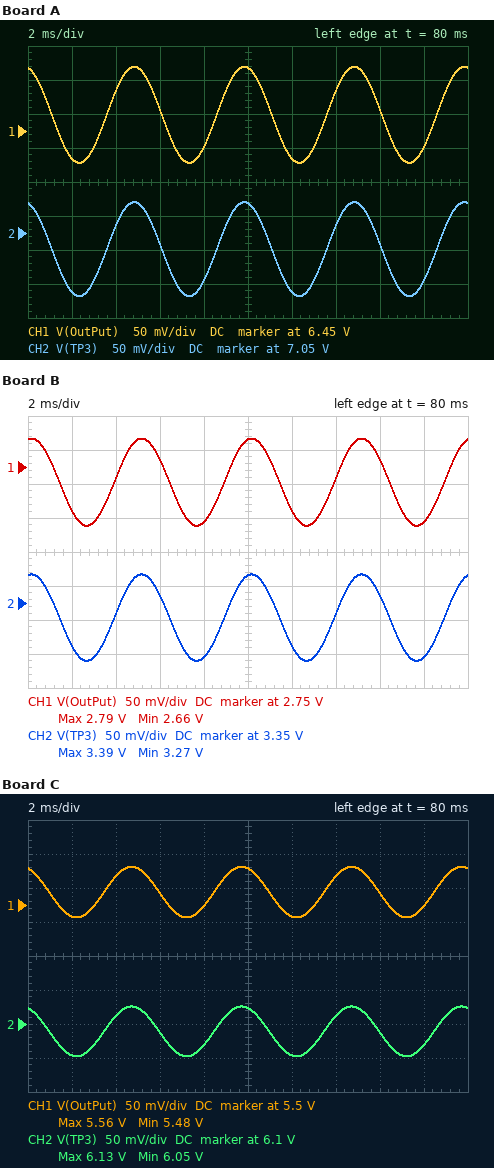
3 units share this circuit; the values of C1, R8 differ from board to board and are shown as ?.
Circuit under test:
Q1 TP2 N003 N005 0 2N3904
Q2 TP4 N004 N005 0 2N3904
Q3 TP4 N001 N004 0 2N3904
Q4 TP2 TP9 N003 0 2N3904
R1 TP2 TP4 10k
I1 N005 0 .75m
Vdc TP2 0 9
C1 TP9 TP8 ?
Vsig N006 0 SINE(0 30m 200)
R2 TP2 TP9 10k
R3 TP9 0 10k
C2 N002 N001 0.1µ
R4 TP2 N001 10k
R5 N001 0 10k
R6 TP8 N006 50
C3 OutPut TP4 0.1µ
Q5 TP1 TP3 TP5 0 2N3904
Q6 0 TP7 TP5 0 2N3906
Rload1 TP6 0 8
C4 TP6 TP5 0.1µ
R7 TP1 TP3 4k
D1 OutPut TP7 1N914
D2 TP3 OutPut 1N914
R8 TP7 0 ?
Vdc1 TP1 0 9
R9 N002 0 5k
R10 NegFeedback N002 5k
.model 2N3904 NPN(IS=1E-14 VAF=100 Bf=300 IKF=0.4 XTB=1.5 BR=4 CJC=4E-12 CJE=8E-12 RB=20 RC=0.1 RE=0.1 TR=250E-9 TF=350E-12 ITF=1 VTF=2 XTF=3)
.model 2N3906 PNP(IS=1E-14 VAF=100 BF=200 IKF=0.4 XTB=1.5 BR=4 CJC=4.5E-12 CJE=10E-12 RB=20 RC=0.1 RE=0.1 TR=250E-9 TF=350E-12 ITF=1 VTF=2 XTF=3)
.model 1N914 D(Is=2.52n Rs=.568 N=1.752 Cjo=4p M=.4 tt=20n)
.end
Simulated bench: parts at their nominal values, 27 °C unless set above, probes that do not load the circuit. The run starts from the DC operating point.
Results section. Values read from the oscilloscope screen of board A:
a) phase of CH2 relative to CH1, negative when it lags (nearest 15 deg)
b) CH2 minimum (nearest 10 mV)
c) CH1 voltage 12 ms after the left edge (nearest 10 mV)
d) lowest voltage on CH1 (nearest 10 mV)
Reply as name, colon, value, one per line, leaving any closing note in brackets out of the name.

phase of CH2 relative to CH1, negative when it lags: 0 deg
CH2 minimum: 6.96 V
CH1 voltage 12 ms after the left edge: 6.41 V
lowest voltage on CH1: 6.40 V
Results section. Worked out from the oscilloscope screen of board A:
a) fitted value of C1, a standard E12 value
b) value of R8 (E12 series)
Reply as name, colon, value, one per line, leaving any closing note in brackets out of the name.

fitted value of C1, a standard E12 value: 56 nF
value of R8: 12 kΩ
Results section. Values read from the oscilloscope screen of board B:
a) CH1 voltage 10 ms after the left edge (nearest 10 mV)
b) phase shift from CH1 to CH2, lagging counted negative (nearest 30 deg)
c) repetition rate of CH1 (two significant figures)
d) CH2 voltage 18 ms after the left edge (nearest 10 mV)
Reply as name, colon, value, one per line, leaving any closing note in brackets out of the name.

CH1 voltage 10 ms after the left edge: 2.79 V
phase shift from CH1 to CH2, lagging counted negative: 0 deg
repetition rate of CH1: 200 Hz
CH2 voltage 18 ms after the left edge: 3.27 V
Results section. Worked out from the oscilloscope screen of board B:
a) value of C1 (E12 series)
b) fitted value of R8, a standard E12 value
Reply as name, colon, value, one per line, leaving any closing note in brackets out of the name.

value of C1: 180 nF
fitted value of R8, a standard E12 value: 1.5 kΩ
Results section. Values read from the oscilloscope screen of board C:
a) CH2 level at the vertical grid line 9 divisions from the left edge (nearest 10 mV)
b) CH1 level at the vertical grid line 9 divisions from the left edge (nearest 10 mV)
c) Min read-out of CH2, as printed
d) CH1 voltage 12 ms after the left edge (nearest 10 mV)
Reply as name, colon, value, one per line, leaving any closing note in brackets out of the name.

CH2 level at the vertical grid line 9 divisions from the left edge: 6.07 V
CH1 level at the vertical grid line 9 divisions from the left edge: 5.50 V
Min read-out of CH2, as printed: 6.05 V
CH1 voltage 12 ms after the left edge: 5.48 V
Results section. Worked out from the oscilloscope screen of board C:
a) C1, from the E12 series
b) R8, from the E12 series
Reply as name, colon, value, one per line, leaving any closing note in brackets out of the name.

C1, from the E12 series: 33 nF
R8, from the E12 series: 6.8 kΩ
